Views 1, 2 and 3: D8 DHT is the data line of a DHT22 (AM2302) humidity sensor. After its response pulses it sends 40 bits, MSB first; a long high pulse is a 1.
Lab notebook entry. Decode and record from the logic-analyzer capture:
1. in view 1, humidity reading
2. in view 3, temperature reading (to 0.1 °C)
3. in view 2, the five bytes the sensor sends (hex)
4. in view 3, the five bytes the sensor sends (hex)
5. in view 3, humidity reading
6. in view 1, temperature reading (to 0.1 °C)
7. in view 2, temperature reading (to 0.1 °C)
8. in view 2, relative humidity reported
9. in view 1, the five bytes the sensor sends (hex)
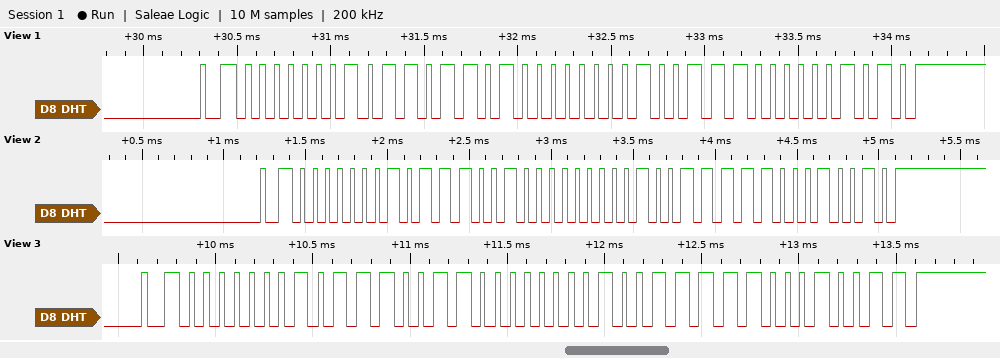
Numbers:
36.5 %
15.9 °C
01 72 00 9F 12
01 73 00 9F 13
37.1 %
15.6 °C
15.9 °C
37.0 %
01 6D 00 9C 0A
